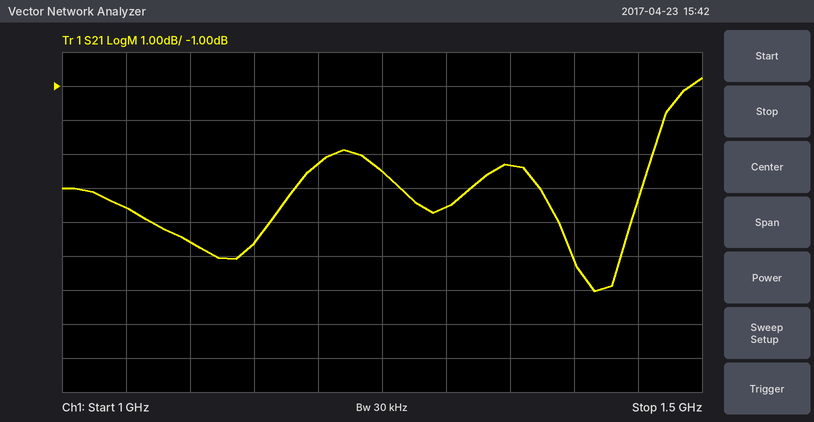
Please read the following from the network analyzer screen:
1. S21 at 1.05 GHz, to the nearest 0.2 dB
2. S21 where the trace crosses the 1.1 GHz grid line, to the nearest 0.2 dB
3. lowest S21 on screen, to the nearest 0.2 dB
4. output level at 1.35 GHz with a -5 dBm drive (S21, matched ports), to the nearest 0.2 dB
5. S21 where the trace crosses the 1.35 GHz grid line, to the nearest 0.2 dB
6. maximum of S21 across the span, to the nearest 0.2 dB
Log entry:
-4.6 dB
-5.6 dB
-7.0 dB
-8.4 dBm
-3.4 dB
-0.8 dB
